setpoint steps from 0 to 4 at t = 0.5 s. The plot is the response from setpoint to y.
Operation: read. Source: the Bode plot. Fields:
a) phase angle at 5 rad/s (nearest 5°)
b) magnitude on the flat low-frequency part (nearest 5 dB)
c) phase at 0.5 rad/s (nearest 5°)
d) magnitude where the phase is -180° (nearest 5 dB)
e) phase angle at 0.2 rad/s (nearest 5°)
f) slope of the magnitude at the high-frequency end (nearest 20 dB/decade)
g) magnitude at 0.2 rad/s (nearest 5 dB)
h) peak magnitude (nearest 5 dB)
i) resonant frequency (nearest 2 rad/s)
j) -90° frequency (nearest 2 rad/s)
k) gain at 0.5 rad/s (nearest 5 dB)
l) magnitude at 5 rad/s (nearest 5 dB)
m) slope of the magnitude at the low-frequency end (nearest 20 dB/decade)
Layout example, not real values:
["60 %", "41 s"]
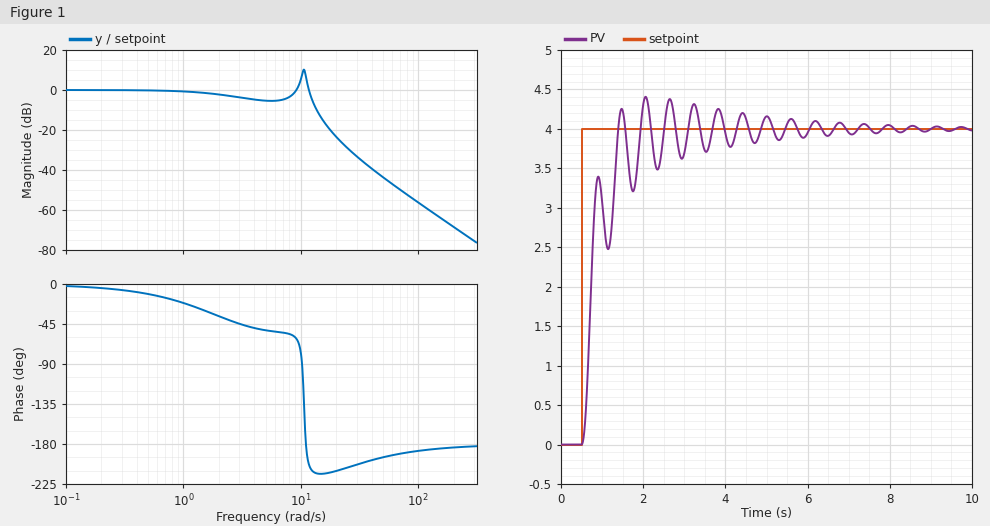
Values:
["-50°", "0 dB", "-10°", "5 dB", "-5°", "-40 dB/decade", "0 dB", "10 dB", "10 rad/s", "10 rad/s", "0 dB", "-5 dB", "0 dB/decade"]
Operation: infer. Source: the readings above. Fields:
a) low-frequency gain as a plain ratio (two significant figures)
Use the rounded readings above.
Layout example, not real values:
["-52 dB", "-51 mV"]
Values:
["1.0"]
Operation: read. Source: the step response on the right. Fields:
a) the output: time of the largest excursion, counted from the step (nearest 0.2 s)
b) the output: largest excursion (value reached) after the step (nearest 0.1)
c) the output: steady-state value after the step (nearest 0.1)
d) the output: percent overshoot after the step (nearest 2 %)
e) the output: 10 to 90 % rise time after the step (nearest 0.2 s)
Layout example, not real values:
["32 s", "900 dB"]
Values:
["1.6 s", "4.4", "4.0", "10 %", "0.8 s"]
